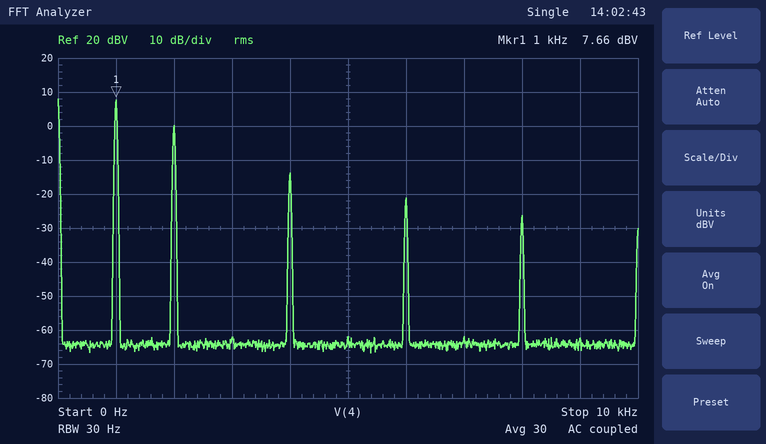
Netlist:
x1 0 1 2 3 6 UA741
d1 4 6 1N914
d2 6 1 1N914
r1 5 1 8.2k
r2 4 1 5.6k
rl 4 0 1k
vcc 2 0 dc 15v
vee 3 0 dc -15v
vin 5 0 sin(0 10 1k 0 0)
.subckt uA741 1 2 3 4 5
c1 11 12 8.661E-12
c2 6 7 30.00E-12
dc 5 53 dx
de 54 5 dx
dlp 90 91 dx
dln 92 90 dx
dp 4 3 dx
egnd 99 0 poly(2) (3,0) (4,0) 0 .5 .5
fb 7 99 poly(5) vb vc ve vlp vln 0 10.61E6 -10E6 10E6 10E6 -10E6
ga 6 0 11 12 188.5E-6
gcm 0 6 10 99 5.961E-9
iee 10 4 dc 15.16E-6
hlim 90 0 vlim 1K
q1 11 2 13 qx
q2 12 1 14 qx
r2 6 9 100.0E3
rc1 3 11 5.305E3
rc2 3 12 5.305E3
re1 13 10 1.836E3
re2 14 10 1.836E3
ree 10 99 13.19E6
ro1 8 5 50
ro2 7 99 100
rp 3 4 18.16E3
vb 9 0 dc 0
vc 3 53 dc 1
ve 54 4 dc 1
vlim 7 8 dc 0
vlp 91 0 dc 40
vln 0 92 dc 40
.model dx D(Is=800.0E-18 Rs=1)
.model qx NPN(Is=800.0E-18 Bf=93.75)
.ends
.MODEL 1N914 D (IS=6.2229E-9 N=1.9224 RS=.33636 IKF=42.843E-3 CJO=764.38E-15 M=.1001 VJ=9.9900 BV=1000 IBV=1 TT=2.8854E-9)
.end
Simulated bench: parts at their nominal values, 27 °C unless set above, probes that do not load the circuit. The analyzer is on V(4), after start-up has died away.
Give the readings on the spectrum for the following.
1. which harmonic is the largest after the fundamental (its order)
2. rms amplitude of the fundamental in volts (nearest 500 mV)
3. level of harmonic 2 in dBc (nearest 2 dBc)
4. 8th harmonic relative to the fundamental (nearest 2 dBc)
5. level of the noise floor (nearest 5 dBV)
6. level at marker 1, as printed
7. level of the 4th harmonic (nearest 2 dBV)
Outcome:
2
2.5 V
-8 dBc
-34 dBc
-65 dBV
7.66 dBV
-14 dBV
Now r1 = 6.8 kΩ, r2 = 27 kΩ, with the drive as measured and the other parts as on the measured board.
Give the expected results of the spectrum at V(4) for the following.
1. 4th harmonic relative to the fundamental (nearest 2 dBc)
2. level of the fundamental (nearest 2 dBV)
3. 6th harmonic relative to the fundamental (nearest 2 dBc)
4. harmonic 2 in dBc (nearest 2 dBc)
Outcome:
-16 dBc
16 dBV
-18 dBc
-16 dBc
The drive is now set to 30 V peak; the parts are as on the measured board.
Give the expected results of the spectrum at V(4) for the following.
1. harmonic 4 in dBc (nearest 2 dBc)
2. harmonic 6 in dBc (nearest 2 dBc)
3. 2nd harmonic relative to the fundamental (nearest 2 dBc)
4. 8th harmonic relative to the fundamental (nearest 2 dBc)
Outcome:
-14 dBc
-24 dBc
-10 dBc
-42 dBc
